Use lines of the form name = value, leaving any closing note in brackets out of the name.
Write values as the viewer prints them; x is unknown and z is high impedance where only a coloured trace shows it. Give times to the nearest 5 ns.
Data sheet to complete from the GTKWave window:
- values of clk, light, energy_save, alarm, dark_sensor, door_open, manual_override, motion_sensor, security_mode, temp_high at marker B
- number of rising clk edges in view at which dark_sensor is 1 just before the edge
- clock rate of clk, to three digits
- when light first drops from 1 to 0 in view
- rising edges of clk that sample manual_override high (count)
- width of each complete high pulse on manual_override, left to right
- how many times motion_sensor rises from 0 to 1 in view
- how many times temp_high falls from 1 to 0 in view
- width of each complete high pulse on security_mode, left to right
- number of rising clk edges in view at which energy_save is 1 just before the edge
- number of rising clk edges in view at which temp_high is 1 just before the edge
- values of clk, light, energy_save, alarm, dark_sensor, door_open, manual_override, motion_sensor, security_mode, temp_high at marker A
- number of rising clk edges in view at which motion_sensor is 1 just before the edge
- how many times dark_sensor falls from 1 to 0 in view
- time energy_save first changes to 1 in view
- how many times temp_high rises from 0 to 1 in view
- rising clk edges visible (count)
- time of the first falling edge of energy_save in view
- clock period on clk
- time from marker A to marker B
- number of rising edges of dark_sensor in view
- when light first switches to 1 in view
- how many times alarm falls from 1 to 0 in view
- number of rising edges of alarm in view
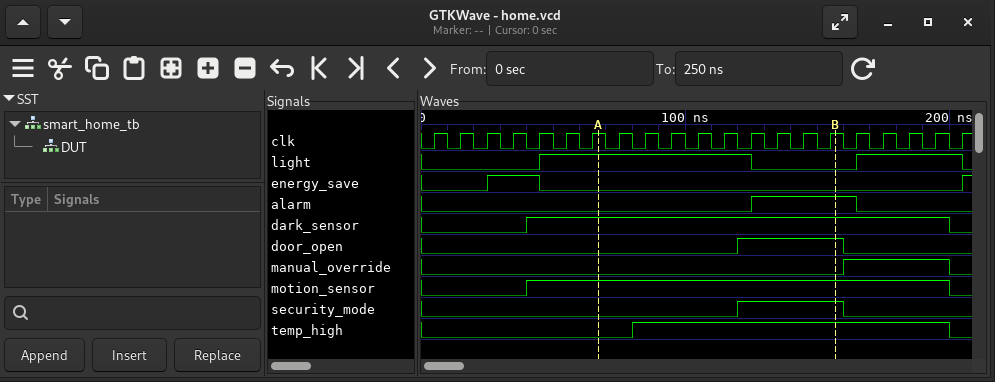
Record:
values of clk, light, energy_save, alarm, dark_sensor, door_open, manual_override, motion_sensor, security_mode, temp_high at marker B = clk=1, light=0, energy_save=0, alarm=1, dark_sensor=1, door_open=1, manual_override=0, motion_sensor=1, security_mode=1, temp_high=1
number of rising clk edges in view at which dark_sensor is 1 just before the edge = 16
clock rate of clk, to three digits = 100 MHz
when light first drops from 1 to 0 in view = 125 ns
rising edges of clk that sample manual_override high = 4
width of each complete high pulse on manual_override, left to right = 40 ns
how many times motion_sensor rises from 0 to 1 in view = 1
how many times temp_high falls from 1 to 0 in view = 1
width of each complete high pulse on security_mode, left to right = 40 ns
number of rising clk edges in view at which energy_save is 1 just before the edge = 2
number of rising clk edges in view at which temp_high is 1 just before the edge = 12
values of clk, light, energy_save, alarm, dark_sensor, door_open, manual_override, motion_sensor, security_mode, temp_high at marker A = clk=1, light=1, energy_save=0, alarm=0, dark_sensor=1, door_open=0, manual_override=0, motion_sensor=1, security_mode=0, temp_high=0
number of rising clk edges in view at which motion_sensor is 1 just before the edge = 16
how many times dark_sensor falls from 1 to 0 in view = 1
time energy_save first changes to 1 in view = 25 ns
how many times temp_high rises from 0 to 1 in view = 1
rising clk edges visible = 21
time of the first falling edge of energy_save in view = 45 ns
clock period on clk = 10 ns
time from marker A to marker B = 90 ns
number of rising edges of dark_sensor in view = 1
when light first switches to 1 in view = 45 ns
how many times alarm falls from 1 to 0 in view = 1
number of rising edges of alarm in view = 1
